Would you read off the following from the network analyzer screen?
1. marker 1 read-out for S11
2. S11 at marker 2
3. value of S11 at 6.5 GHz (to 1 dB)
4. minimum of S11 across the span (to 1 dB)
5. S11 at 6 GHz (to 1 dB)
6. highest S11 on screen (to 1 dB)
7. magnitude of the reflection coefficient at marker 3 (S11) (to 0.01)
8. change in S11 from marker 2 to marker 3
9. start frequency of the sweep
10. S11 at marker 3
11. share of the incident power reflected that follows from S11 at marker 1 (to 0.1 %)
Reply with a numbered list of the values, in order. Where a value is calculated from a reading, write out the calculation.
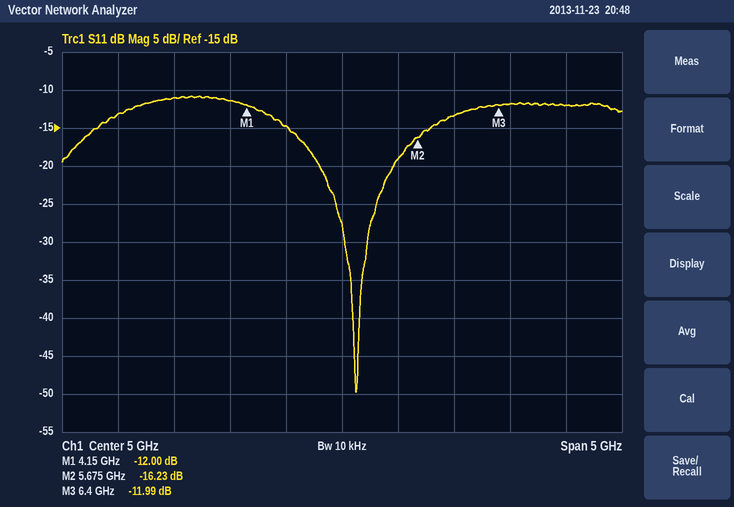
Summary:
1. -12.00 dB
2. -16.23 dB
3. -12 dB
4. -50 dB
5. -13 dB
6. -11 dB
7. 10^(-11.99/20) ≈ 0.25
8. -11.99 − (-16.23) = 4.24 dB
9. 2.5 GHz
10. -11.99 dB
11. 10^(-12/10) ≈ 6.3 %
